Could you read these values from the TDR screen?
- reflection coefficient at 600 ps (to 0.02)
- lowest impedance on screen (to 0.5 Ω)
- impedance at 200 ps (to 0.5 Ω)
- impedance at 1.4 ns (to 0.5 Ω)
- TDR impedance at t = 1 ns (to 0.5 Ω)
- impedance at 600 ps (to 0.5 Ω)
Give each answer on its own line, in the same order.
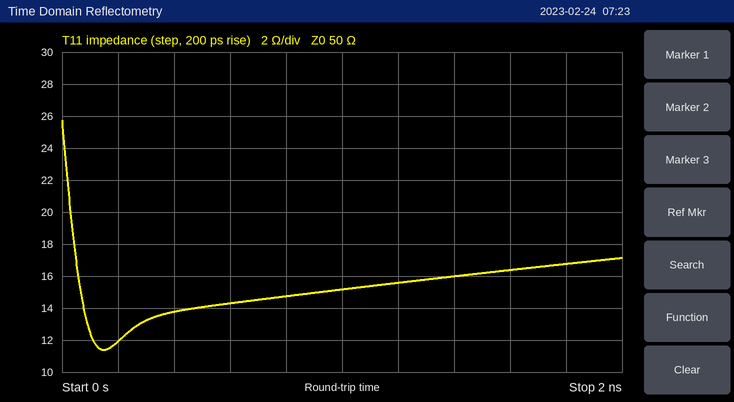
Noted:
-0.56
11.5 Ω
12.0 Ω
16.0 Ω
15.0 Ω
14.5 Ω
